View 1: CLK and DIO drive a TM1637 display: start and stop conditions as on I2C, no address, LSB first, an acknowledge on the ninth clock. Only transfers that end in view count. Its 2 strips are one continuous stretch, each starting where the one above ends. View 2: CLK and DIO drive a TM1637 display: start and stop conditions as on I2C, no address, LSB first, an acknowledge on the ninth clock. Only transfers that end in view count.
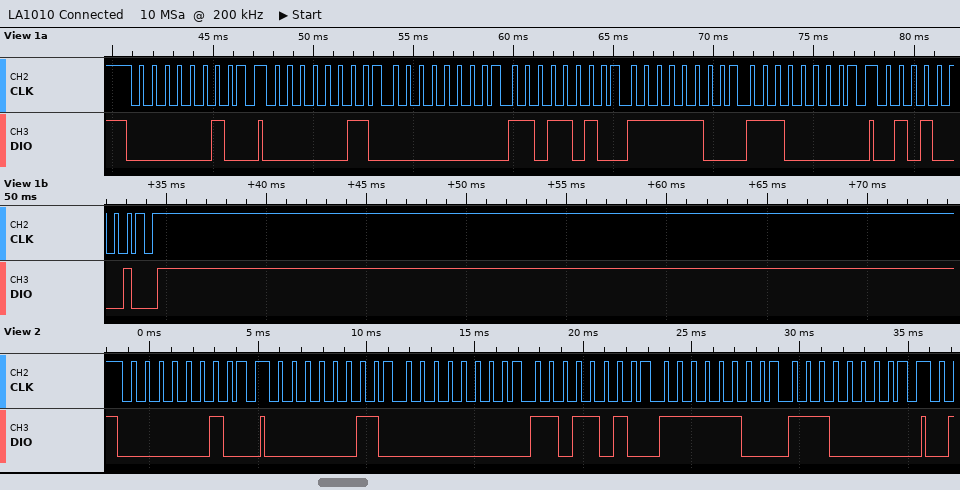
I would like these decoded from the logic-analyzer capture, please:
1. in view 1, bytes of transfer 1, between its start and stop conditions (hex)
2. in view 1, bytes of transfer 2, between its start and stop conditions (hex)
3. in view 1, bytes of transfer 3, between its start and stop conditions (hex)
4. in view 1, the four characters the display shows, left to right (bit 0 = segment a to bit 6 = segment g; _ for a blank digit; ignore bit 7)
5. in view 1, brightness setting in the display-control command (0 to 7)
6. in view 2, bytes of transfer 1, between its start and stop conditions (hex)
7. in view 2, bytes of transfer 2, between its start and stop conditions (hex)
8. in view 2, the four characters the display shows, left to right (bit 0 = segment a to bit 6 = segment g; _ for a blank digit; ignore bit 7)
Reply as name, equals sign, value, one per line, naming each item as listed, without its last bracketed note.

in view 1, bytes of transfer 1, between its start and stop conditions = 40
in view 1, bytes of transfer 2, between its start and stop conditions = C0 00 5B 3F 07
in view 1, bytes of transfer 3, between its start and stop conditions = 8A
in view 1, the four characters the display shows, left to right = _207
in view 1, brightness setting in the display-control command = 2
in view 2, bytes of transfer 1, between its start and stop conditions = 40
in view 2, bytes of transfer 2, between its start and stop conditions = C0 00 5B 3F 07
in view 2, the four characters the display shows, left to right = _207
